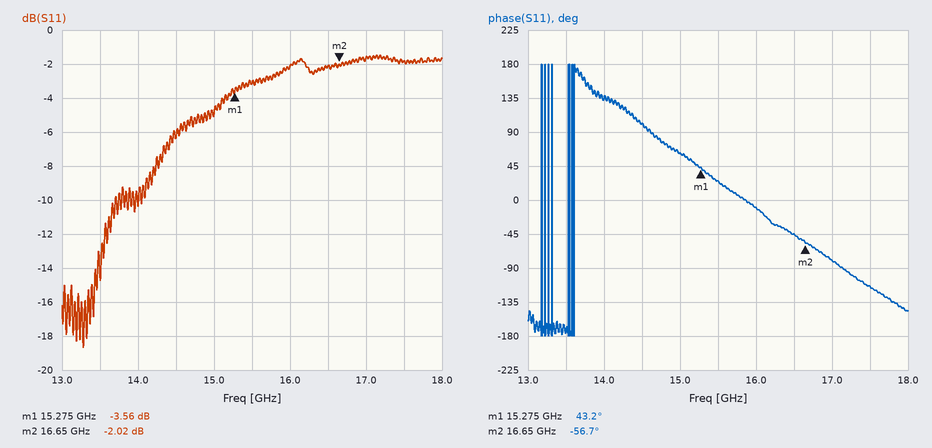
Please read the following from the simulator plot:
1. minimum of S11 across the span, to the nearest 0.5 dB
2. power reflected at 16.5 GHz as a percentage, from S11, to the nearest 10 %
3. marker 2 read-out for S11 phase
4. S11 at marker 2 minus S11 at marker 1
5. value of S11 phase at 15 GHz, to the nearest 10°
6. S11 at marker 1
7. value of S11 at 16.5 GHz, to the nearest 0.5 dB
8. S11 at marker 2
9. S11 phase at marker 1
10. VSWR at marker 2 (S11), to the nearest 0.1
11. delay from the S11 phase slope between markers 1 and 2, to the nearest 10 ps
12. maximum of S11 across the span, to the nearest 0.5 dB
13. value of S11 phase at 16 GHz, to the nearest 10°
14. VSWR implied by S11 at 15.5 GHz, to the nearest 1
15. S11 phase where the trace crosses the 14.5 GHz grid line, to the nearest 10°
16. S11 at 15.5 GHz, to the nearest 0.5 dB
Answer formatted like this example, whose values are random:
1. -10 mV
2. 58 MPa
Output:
1. -18.5 dB
2. 60 %
3. -56.7°
4. 1.54 dB
5. 60°
6. -3.56 dB
7. -2.0 dB
8. -2.02 dB
9. 43.2°
10. 8.6
11. 200 ps
12. -1.5 dB
13. -10°
14. 6
15. 100°
16. -3.0 dB
